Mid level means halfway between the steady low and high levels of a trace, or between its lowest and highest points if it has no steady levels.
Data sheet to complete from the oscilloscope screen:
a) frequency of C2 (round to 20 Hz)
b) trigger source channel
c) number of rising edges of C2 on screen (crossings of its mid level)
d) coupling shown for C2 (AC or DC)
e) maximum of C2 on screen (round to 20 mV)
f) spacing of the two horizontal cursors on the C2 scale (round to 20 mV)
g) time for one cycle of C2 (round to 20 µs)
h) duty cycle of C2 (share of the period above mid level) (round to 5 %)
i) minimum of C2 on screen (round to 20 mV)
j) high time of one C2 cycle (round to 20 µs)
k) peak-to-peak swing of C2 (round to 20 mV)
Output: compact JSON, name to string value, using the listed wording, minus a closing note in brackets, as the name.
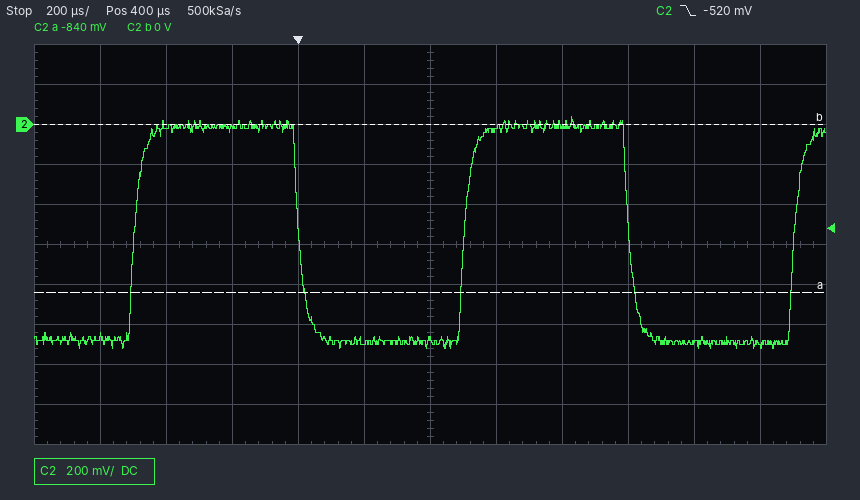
{"frequency of C2": "1.00 kHz", "trigger source channel": "C2", "number of rising edges of C2 on screen": "3", "coupling shown for C2": "DC", "maximum of C2 on screen": "40 mV", "spacing of the two horizontal cursors on the C2 scale": "840 mV", "time for one cycle of C2": "1.00 ms", "duty cycle of C2 (share of the period above mid level)": "50 %", "minimum of C2 on screen": "-1.12 V", "high time of one C2 cycle": "500 µs", "peak-to-peak swing of C2": "1.16 V"}
